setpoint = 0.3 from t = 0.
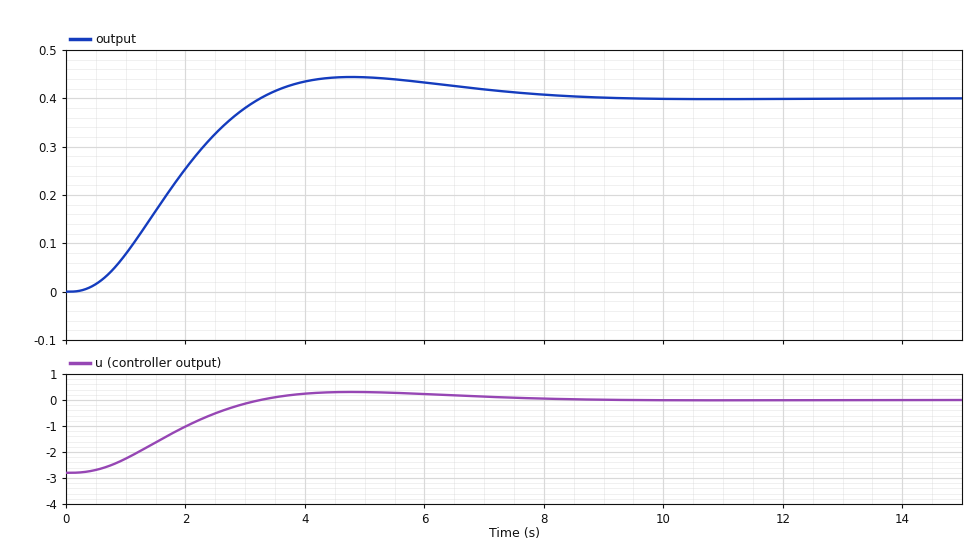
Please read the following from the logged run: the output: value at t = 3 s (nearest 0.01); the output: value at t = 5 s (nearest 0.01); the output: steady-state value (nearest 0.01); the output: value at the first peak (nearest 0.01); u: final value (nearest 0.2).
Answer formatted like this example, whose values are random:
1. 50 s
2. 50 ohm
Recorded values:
1. 0.38
2. 0.44
3. 0.40
4. 0.44
5. 0.0
